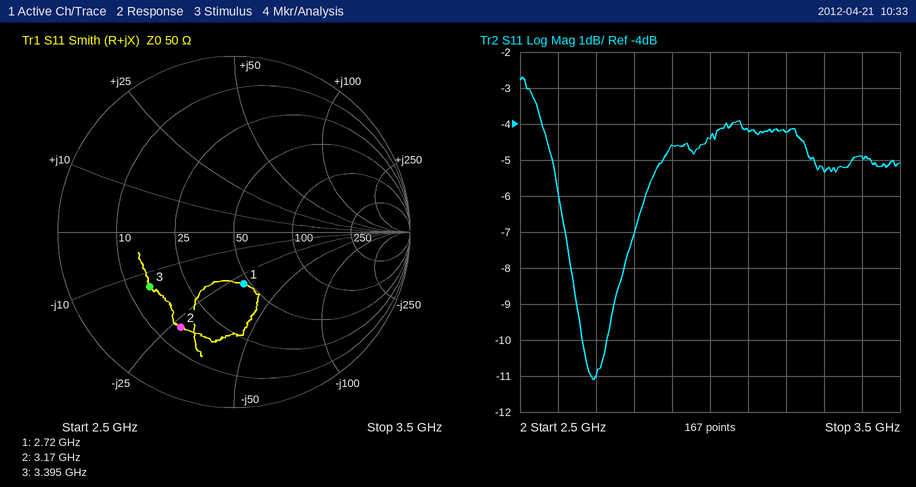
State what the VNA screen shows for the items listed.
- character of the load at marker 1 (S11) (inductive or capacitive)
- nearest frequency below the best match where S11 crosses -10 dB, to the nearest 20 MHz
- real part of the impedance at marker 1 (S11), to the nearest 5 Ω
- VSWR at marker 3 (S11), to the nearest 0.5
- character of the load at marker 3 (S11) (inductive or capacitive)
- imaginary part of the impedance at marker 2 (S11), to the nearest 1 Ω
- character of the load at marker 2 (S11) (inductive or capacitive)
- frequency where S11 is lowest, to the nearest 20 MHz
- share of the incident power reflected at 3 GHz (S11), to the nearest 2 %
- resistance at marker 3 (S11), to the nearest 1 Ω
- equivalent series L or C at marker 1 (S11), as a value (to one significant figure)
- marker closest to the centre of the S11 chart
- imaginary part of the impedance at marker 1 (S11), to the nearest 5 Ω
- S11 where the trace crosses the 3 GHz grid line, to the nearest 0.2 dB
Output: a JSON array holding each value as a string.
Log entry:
["capacitive", "2.66 GHz", "45 Ω", "3.5", "capacitive", "-27 Ω", "capacitive", "2.70 GHz", "36 %", "15 Ω", "2 pF", "marker 1", "-30 Ω", "-4.4 dB"]
